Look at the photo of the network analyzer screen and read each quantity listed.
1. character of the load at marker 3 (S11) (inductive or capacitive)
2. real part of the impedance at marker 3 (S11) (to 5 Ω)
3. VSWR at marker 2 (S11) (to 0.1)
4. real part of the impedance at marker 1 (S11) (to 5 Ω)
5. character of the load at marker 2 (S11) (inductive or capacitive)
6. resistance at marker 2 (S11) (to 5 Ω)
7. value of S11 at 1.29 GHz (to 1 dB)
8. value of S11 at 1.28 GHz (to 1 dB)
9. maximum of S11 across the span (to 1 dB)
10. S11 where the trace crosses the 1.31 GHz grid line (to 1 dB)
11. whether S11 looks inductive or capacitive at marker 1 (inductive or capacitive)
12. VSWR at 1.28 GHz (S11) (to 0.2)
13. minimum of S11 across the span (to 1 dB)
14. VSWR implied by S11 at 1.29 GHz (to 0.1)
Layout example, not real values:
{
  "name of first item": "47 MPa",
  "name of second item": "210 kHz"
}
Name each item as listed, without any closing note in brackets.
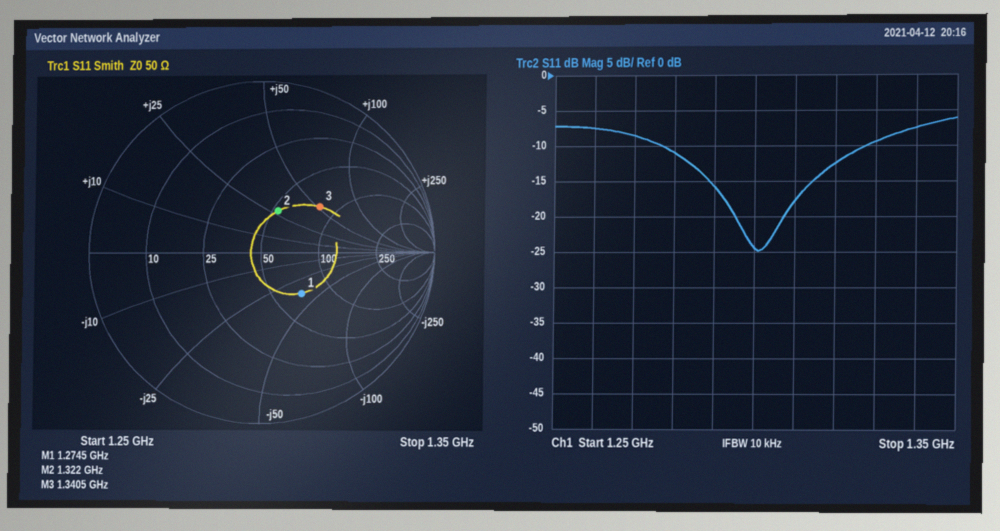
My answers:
{
  "character of the load at marker 3 (S11)": "inductive",
  "real part of the impedance at marker 3 (S11)": "80 Ω",
  "VSWR at marker 2 (S11)": "1.7",
  "real part of the impedance at marker 1 (S11)": "70 Ω",
  "character of the load at marker 2 (S11)": "inductive",
  "resistance at marker 2 (S11)": "55 Ω",
  "value of S11 at 1.29 GHz": "-16 dB",
  "value of S11 at 1.28 GHz": "-11 dB",
  "maximum of S11 across the span": "-6 dB",
  "S11 where the trace crosses the 1.31 GHz grid line": "-18 dB",
  "whether S11 looks inductive or capacitive at marker 1": "capacitive",
  "VSWR at 1.28 GHz (S11)": "1.8",
  "minimum of S11 across the span": "-25 dB",
  "VSWR implied by S11 at 1.29 GHz": "1.4"
}
